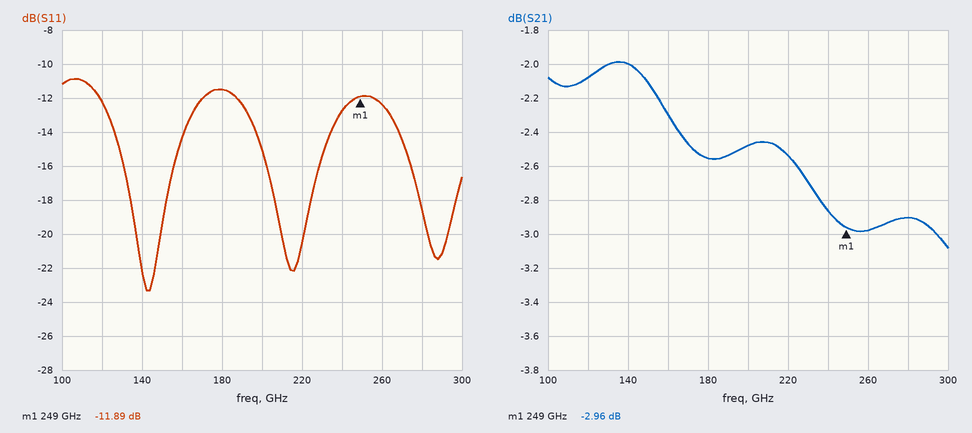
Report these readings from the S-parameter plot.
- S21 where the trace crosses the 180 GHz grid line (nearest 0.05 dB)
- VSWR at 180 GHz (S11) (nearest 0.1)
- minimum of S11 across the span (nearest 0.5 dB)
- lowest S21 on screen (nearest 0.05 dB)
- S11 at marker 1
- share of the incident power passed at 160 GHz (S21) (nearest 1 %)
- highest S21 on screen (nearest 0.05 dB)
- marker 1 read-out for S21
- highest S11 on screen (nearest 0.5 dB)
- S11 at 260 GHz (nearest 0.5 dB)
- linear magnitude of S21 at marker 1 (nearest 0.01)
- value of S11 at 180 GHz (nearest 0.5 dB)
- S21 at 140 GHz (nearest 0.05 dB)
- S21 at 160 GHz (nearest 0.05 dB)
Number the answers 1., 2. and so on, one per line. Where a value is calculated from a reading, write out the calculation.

1. -2.55 dB
2. |Γ| = 10^(-11.5/20) = 0.2661; VSWR = (1 + 0.2661)/(1 − 0.2661) ≈ 1.7
3. -23.5 dB
4. -3.10 dB
5. -11.89 dB
6. 10^(-2.3/10) ≈ 59 %
7. -2.00 dB
8. -2.96 dB
9. -11.0 dB
10. -12.5 dB
11. 10^(-2.96/20) ≈ 0.71
12. -11.5 dB
13. -2.00 dB
14. -2.30 dB
